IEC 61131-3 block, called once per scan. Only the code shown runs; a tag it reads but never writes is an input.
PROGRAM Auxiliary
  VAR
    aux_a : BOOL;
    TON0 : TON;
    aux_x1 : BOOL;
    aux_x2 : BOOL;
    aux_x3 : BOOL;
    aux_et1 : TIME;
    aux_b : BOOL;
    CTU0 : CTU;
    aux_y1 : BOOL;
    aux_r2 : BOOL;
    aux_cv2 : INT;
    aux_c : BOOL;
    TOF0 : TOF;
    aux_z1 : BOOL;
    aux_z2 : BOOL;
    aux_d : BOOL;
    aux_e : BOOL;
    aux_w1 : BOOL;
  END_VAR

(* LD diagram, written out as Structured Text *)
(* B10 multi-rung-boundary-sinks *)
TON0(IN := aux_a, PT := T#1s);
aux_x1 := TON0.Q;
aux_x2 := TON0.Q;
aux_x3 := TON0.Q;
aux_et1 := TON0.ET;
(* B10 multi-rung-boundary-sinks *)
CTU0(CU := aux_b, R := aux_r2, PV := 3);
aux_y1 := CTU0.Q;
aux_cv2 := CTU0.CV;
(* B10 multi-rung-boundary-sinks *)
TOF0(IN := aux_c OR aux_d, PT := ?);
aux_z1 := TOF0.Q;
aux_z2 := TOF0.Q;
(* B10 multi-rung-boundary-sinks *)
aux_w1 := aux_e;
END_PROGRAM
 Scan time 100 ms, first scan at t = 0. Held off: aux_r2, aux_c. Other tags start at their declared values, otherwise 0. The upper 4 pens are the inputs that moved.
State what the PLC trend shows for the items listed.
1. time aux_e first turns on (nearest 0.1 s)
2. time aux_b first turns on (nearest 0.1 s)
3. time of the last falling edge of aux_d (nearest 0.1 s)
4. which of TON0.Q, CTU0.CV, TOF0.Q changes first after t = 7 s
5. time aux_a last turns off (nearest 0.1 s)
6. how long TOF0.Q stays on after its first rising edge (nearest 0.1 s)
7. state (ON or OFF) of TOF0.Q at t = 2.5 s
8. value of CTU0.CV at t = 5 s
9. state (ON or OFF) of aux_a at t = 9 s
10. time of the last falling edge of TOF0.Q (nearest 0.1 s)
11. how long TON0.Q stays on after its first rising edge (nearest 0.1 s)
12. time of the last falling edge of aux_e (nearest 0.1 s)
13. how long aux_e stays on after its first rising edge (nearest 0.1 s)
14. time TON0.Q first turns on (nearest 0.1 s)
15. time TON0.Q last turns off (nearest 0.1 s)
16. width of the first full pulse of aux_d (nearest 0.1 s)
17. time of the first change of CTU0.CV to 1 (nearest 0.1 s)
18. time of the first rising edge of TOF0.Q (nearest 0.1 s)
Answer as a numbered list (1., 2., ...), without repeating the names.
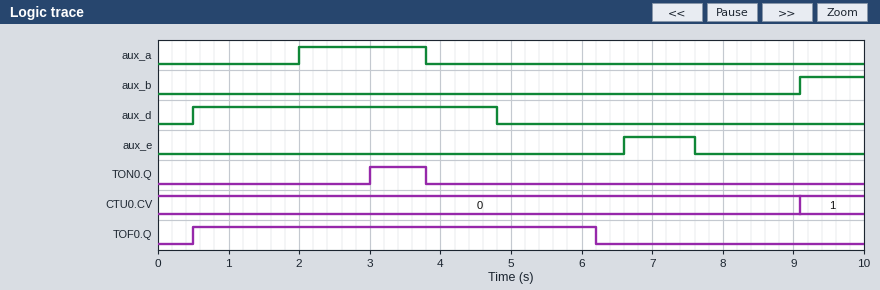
1. 6.6 s
2. 9.1 s
3. 4.8 s
4. CTU0.CV
5. 3.8 s
6. 5.7 s
7. ON
8. 0
9. OFF
10. 6.2 s
11. 0.8 s
12. 7.6 s
13. 1.0 s
14. 3.0 s
15. 3.8 s
16. 4.3 s
17. 9.1 s
18. 0.5 s
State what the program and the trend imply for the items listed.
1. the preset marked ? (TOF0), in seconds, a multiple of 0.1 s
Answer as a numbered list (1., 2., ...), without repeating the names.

1. 1.4 s
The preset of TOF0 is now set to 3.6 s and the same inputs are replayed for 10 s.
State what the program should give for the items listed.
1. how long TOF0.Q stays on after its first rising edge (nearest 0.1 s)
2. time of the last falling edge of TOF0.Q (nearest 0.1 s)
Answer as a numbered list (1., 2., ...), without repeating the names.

1. 7.9 s
2. 8.4 s
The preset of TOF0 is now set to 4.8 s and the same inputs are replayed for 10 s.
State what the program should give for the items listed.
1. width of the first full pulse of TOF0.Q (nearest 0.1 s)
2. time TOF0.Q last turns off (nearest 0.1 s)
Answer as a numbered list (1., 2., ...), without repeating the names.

1. 9.1 s
2. 9.6 s
